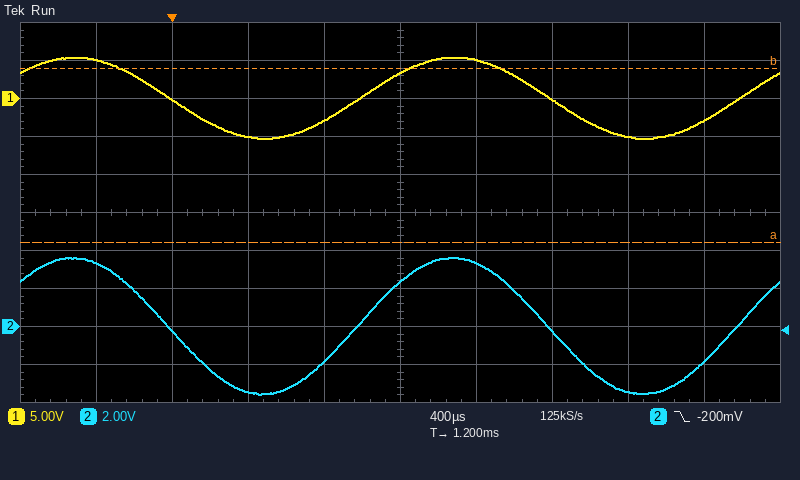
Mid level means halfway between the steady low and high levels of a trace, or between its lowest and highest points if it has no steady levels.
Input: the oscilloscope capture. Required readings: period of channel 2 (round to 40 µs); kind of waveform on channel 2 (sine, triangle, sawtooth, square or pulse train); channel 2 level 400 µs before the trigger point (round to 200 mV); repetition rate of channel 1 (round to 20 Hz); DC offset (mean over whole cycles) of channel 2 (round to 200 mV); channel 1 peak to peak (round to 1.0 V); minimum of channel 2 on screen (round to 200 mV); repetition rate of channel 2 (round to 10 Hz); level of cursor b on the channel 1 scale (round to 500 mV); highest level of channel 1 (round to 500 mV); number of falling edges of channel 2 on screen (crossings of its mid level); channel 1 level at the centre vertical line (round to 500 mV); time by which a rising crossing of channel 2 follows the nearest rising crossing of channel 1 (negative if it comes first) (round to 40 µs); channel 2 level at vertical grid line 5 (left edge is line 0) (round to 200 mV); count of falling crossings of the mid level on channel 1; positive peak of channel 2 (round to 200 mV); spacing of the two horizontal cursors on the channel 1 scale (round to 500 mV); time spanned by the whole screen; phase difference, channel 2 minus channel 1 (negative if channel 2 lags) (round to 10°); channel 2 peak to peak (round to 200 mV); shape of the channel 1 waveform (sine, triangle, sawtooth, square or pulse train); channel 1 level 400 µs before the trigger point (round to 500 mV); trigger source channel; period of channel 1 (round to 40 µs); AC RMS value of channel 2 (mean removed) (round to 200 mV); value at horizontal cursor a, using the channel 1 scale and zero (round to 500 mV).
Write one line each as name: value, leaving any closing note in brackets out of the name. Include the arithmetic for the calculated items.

period of channel 2: 2.00 ms
kind of waveform on channel 2: sine
channel 2 level 400 µs before the trigger point: 3.4 V
repetition rate of channel 1: 1 / 2.00 ms ≈ 500 Hz
DC offset (mean over whole cycles) of channel 2: (3.6 V + (-3.6 V)) / 2 ≈ 0.0 V
channel 1 peak to peak: 11.0 V
minimum of channel 2 on screen: -3.6 V
repetition rate of channel 2: 1 / 2.00 ms ≈ 500 Hz
level of cursor b on the channel 1 scale: 4.0 V
highest level of channel 1: 5.5 V
number of falling edges of channel 2 on screen: 2
channel 1 level at the centre vertical line: 3.5 V
time by which a rising crossing of channel 2 follows the nearest rising crossing of channel 1 (negative if it comes first): 0 µs
channel 2 level at vertical grid line 5 (left edge is line 0): 2.4 V
count of falling crossings of the mid level on channel 1: 2
positive peak of channel 2: 3.6 V
spacing of the two horizontal cursors on the channel 1 scale: 23.0 V
time spanned by the whole screen: 4 ms
phase difference, channel 2 minus channel 1 (negative if channel 2 lags): −360° × (0 µs) / 2.00 ms ≈ 0°
channel 2 peak to peak: 3.6 V − (-3.6 V) = 7.2 V
shape of the channel 1 waveform: sine
channel 1 level 400 µs before the trigger point: 5.0 V
trigger source channel: channel 2
period of channel 1: 2.00 ms
AC RMS value of channel 2 (mean removed): 7.2 V / (2√2) ≈ 2.6 V
value at horizontal cursor a, using the channel 1 scale and zero: -19.0 V
